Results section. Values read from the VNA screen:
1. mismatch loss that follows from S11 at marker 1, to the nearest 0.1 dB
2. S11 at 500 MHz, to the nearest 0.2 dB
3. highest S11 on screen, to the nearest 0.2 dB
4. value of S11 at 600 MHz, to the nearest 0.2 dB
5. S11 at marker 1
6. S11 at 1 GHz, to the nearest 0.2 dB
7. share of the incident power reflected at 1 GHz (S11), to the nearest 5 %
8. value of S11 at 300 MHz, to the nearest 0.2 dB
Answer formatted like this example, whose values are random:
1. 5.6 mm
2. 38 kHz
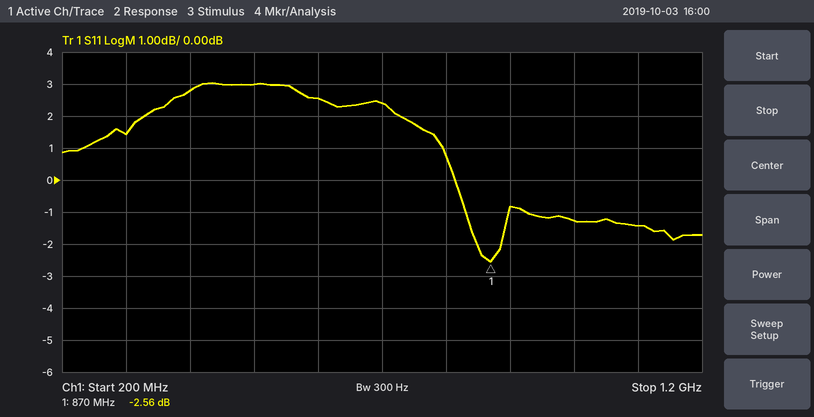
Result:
1. 3.5 dB
2. 3.0 dB
3. 3.0 dB
4. 2.6 dB
5. -2.56 dB
6. -1.2 dB
7. 75 %
8. 1.4 dB
